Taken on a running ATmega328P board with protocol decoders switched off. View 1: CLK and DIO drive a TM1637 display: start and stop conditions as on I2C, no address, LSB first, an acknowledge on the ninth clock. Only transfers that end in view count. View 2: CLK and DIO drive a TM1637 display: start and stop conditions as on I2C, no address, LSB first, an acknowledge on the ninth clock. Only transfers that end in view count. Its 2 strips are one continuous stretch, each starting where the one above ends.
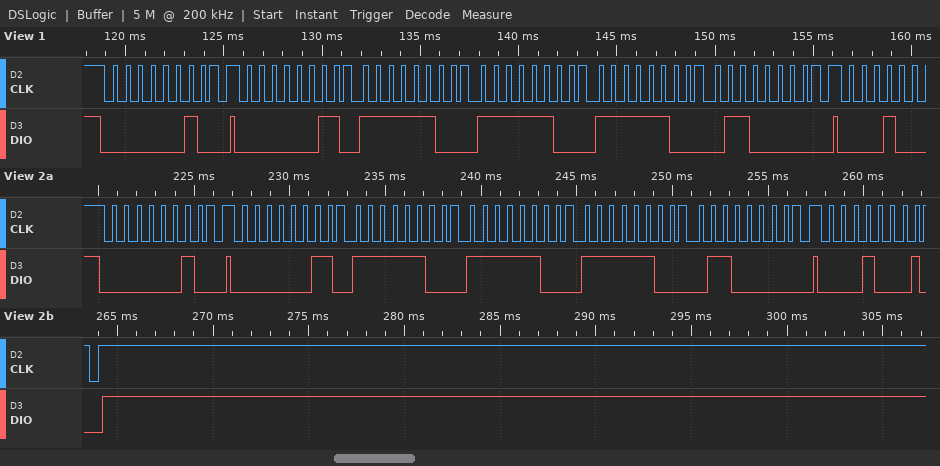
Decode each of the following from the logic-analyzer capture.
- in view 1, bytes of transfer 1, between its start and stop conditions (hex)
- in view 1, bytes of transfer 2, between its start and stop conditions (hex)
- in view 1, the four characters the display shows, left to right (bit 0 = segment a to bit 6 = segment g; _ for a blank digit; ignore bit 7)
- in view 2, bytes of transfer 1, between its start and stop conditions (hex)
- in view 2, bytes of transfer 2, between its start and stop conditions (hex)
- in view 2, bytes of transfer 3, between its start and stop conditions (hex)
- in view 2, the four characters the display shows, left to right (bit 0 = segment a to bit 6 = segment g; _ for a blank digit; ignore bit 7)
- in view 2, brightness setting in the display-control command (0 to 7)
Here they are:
40
C0 3F 3F 3F 06
0001
40
C0 3F 3F 3F 06
88
0001
0
